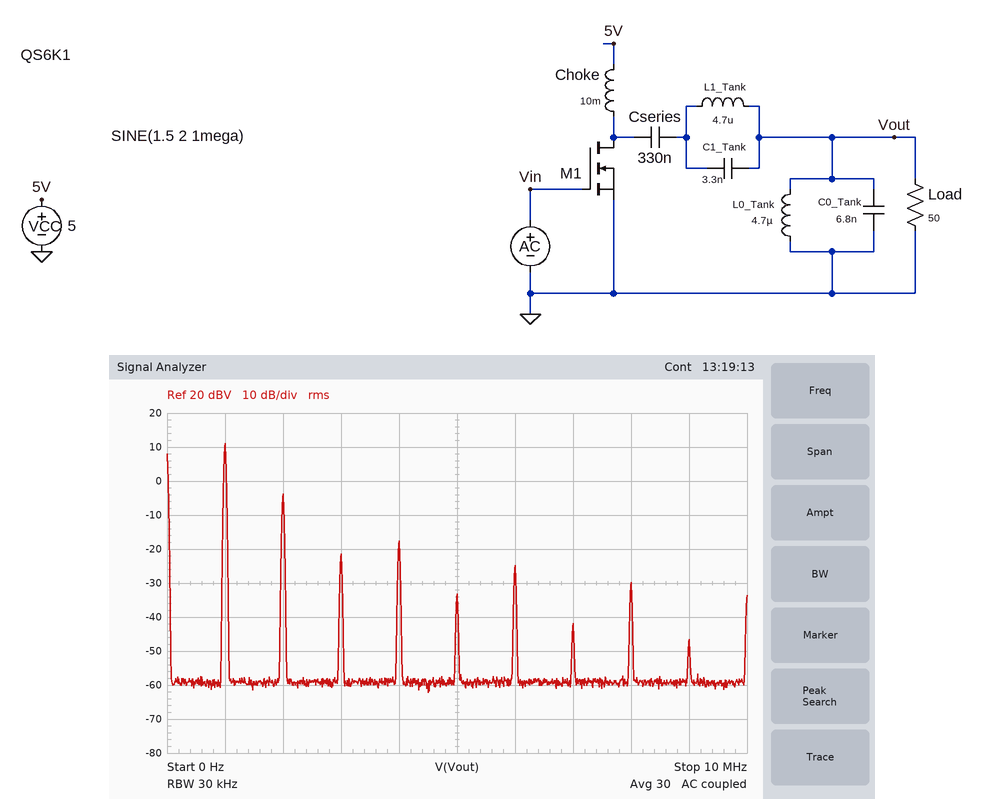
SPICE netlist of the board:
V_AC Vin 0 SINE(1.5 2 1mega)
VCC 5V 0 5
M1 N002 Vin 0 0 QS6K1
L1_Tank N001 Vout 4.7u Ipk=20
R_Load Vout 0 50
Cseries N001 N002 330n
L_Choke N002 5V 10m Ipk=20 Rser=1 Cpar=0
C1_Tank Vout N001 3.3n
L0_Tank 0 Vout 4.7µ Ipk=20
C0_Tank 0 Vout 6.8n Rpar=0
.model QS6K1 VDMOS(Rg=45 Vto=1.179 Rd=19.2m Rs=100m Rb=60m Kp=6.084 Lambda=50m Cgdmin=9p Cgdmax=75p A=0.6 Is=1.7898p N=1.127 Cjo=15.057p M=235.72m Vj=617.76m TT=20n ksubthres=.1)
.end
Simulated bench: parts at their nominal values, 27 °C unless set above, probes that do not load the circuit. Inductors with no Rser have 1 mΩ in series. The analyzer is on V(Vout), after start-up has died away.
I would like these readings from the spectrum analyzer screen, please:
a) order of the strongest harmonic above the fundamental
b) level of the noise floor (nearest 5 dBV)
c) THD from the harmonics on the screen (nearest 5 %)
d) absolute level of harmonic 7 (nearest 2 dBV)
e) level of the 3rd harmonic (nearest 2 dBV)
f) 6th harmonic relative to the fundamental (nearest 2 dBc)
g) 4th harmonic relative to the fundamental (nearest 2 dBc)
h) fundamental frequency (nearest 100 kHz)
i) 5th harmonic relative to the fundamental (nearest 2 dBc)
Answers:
2
-60 dBV
20 %
-42 dBV
-22 dBV
-36 dBc
-28 dBc
1.0 MHz
-44 dBc
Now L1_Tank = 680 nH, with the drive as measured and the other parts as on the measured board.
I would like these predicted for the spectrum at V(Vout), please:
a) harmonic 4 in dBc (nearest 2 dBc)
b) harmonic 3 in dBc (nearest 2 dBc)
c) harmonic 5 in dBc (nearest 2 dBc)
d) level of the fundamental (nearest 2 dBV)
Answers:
-26 dBc
-22 dBc
-46 dBc
14 dBV
